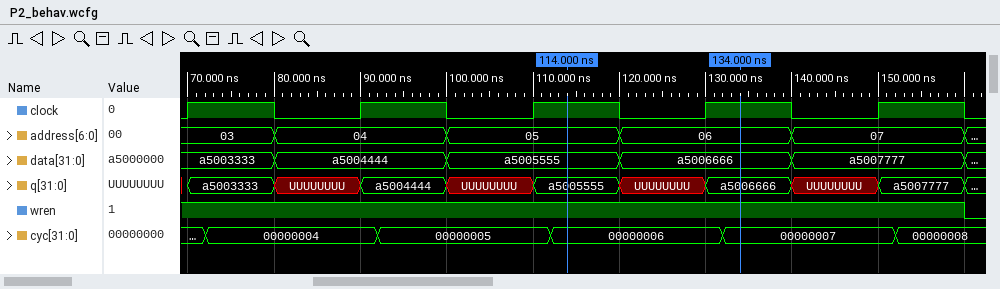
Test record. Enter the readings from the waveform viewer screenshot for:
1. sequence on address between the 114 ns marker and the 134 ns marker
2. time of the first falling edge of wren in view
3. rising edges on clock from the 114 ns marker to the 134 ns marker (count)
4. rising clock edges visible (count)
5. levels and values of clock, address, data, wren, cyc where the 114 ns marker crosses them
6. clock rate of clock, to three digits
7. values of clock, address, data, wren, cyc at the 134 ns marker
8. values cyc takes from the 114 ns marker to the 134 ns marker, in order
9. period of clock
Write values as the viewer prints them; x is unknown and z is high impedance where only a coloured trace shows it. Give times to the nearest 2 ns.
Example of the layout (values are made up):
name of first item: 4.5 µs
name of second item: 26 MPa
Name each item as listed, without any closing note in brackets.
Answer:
sequence on address between the 114 ns marker and the 134 ns marker: 05, 06
time of the first falling edge of wren in view: 160 ns
rising edges on clock from the 114 ns marker to the 134 ns marker: 1
rising clock edges visible: 5
levels and values of clock, address, data, wren, cyc where the 114 ns marker crosses them: clock=1, address=05, data=a5005555, wren=1, cyc=00000006
clock rate of clock, to three digits: 50.0 MHz
values of clock, address, data, wren, cyc at the 134 ns marker: clock=1, address=06, data=a5006666, wren=1, cyc=00000007
values cyc takes from the 114 ns marker to the 134 ns marker, in order: 00000006, 00000007
period of clock: 20 ns
